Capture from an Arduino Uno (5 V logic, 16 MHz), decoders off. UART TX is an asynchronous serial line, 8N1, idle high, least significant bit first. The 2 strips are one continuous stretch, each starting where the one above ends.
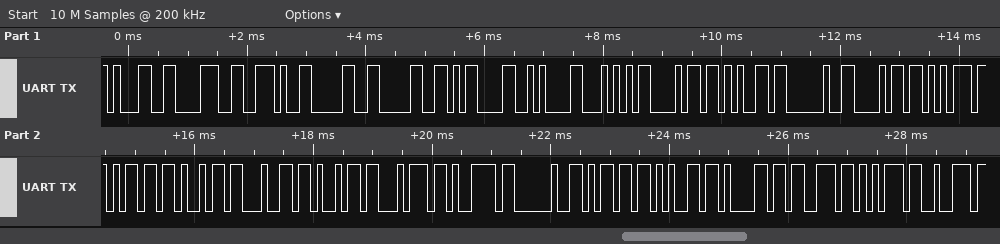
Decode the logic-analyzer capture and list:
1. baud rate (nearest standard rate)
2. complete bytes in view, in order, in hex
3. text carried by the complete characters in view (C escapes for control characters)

9600 baud
31 38 2E 30 30 0D 0A 54 68 65 20 68 75 6D 69 64 69 74 79 20 6D 65 61 73 75 72
"18.00\r\nThe humidity measur"
